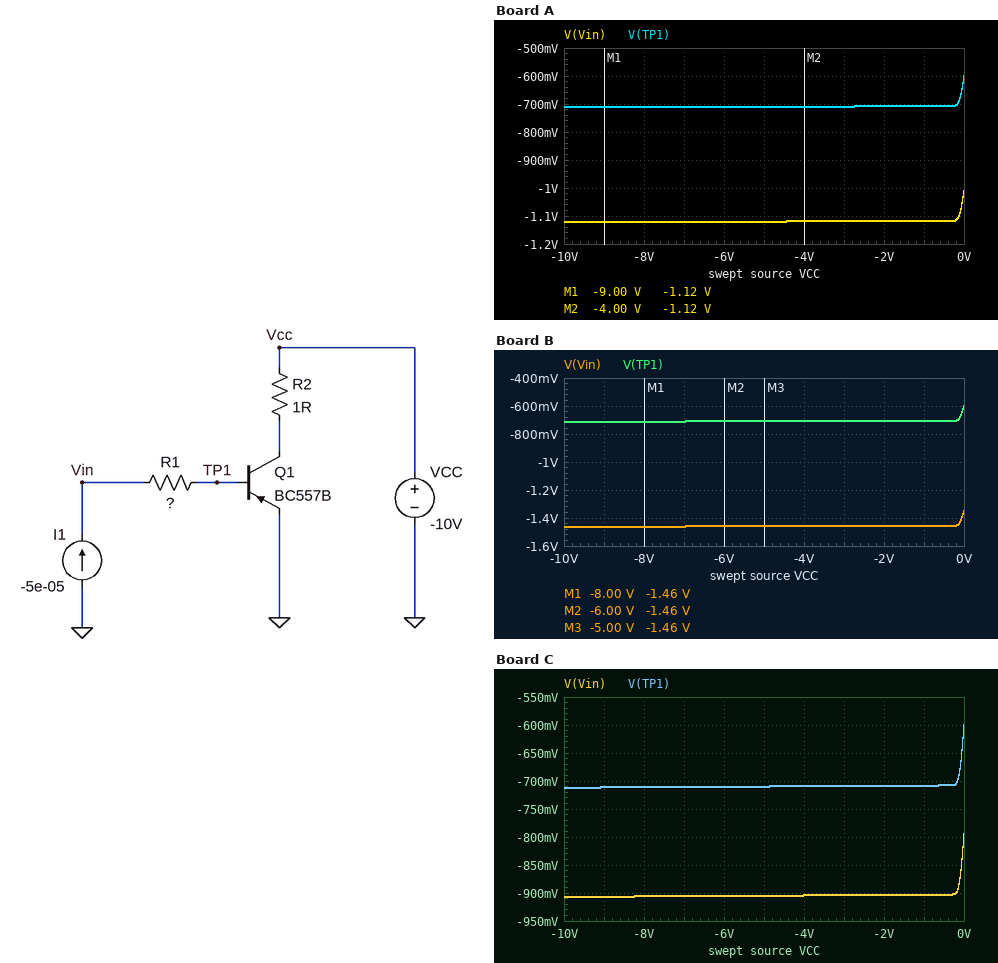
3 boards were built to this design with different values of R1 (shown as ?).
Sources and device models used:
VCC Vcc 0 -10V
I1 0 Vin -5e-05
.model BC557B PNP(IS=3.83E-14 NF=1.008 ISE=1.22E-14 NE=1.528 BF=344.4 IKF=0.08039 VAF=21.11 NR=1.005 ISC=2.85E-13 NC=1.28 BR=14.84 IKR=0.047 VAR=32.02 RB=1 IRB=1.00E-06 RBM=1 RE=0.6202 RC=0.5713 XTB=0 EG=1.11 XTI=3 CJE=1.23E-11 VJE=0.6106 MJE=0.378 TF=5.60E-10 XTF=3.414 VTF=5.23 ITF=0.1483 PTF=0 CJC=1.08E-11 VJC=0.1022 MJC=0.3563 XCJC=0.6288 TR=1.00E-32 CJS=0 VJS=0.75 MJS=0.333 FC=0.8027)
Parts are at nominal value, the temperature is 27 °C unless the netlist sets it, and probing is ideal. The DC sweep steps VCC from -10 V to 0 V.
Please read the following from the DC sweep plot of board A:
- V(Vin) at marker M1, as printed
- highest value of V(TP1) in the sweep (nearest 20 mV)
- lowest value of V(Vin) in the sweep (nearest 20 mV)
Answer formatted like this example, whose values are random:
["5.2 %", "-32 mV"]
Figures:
["-1.12 V", "-600 mV", "-1.12 V"]
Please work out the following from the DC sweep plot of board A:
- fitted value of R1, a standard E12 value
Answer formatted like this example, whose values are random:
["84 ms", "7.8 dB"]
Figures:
["8.2 kΩ"]
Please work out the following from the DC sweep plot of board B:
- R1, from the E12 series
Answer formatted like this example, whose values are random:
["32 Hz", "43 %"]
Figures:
["15 kΩ"]
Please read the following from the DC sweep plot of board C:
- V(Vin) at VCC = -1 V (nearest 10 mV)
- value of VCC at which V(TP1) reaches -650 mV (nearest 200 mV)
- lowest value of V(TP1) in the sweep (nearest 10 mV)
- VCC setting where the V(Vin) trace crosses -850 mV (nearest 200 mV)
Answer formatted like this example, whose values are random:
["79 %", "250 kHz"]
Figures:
["-900 mV", "0 V", "-710 mV", "0 V"]
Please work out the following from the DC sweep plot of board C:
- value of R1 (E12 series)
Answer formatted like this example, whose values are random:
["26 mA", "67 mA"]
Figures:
["3.9 kΩ"]
